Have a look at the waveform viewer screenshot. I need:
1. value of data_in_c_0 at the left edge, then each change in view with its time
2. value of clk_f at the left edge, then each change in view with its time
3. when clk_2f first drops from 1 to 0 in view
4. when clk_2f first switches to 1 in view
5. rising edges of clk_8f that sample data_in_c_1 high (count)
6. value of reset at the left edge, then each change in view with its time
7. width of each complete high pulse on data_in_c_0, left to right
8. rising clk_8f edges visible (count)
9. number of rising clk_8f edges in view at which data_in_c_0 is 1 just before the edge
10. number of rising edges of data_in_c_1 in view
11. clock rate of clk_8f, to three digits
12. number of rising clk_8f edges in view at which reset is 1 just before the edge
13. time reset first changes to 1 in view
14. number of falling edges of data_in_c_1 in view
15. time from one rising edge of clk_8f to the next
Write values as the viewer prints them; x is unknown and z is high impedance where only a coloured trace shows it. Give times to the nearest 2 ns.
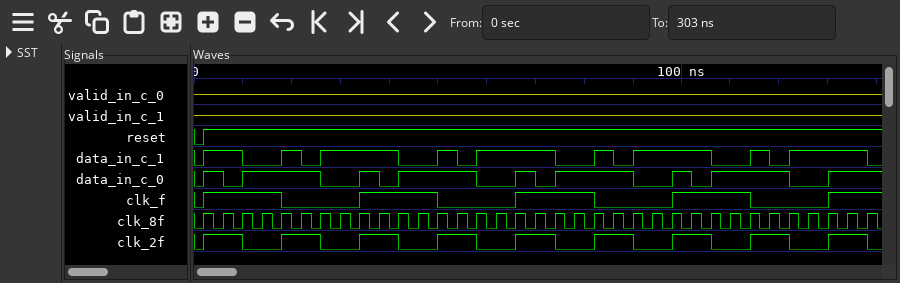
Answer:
0, 1 at 2 ns, 0 at 6 ns, 1 at 10 ns, 0 at 26 ns, 1 at 34 ns, 0 at 38 ns, 1 at 42 ns, 0 at 58 ns, 1 at 66 ns, 0 at 70 ns, 1 at 74 ns, 0 at 90 ns, 1 at 98 ns, 0 at 102 ns, 1 at 106 ns, 0 at 122 ns, 1 at 130 ns
0, 1 at 2 ns, 0 at 18 ns, 1 at 34 ns, 0 at 50 ns, 1 at 66 ns, 0 at 82 ns, 1 at 98 ns, 0 at 114 ns, 1 at 130 ns
10 ns
2 ns
22
0, 1 at 2 ns
4 ns, 16 ns, 4 ns, 16 ns, 4 ns, 16 ns, 4 ns, 16 ns
35
22
9
250 MHz
34
2 ns
9
4 ns
